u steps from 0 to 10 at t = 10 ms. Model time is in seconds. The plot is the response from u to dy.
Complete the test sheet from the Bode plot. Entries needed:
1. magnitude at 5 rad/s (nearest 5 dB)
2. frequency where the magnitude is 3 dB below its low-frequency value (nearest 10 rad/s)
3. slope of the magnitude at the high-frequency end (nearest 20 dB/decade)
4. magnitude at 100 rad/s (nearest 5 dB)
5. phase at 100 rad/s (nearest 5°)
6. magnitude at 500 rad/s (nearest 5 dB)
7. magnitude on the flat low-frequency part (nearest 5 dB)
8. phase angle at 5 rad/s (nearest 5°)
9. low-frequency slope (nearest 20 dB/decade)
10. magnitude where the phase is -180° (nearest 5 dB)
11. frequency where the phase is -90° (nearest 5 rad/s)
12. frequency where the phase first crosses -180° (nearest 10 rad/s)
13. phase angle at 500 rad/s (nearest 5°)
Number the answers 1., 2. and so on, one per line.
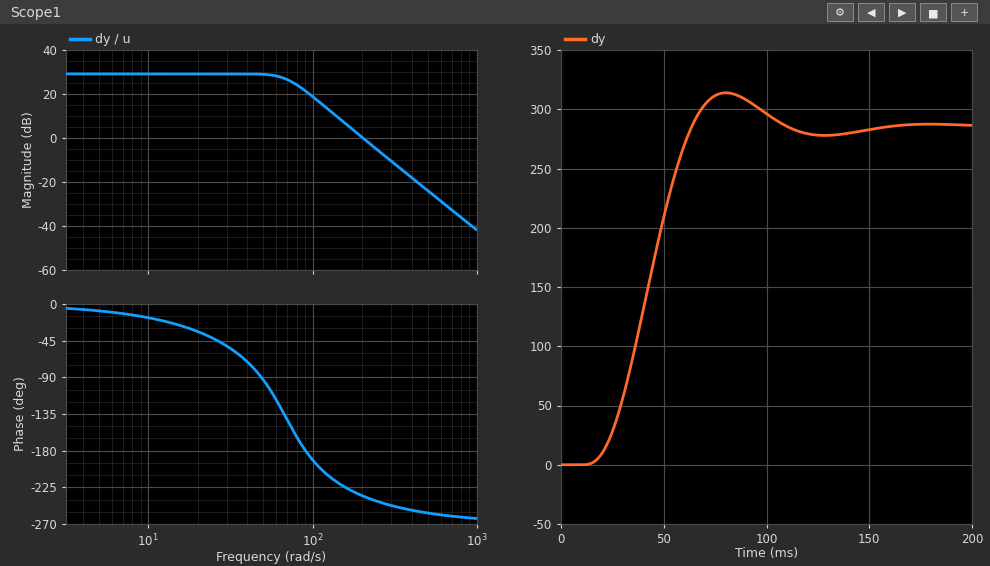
1. 30 dB
2. 70 rad/s
3. -60 dB/decade
4. 20 dB
5. -190°
6. -25 dB
7. 30 dB
8. -10°
9. 0 dB/decade
10. 20 dB
11. 50 rad/s
12. 90 rad/s
13. -255°
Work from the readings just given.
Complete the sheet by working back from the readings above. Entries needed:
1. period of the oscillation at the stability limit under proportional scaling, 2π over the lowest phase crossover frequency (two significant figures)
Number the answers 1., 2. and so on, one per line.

1. 0.070 s
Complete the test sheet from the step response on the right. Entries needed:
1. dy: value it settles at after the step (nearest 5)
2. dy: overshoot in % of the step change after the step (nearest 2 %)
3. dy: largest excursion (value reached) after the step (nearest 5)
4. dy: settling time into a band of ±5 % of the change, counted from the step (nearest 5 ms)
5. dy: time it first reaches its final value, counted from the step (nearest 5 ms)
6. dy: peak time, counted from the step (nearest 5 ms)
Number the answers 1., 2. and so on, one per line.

1. 285
2. 10 %
3. 315
4. 85 ms
5. 55 ms
6. 70 ms
